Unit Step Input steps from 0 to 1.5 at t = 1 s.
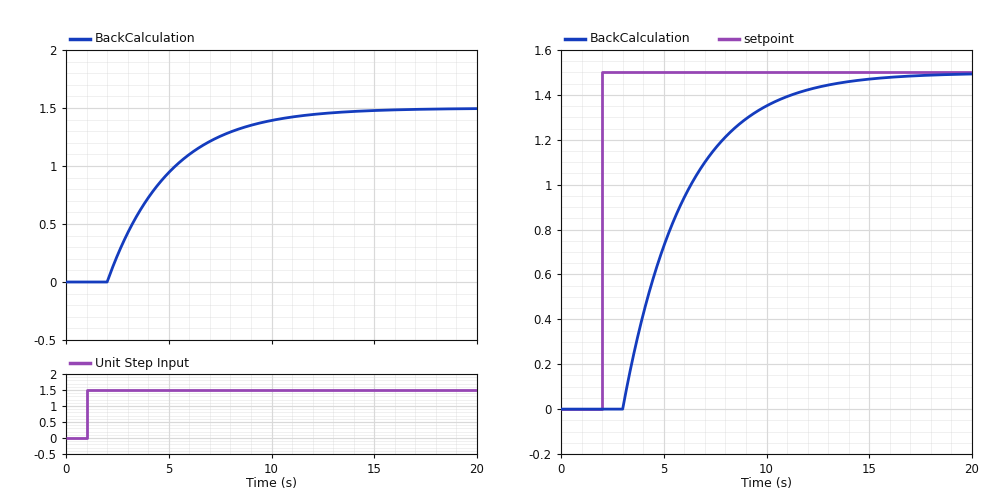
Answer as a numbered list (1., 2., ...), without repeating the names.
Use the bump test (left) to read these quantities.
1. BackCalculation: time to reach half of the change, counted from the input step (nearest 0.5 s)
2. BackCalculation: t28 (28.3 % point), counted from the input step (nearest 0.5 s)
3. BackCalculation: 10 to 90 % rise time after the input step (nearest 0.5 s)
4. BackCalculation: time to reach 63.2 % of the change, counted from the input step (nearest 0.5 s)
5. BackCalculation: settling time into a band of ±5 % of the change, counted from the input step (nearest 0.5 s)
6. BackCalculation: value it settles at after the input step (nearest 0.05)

1. 3.0 s
2. 2.0 s
3. 6.5 s
4. 4.0 s
5. 10.0 s
6. 1.50
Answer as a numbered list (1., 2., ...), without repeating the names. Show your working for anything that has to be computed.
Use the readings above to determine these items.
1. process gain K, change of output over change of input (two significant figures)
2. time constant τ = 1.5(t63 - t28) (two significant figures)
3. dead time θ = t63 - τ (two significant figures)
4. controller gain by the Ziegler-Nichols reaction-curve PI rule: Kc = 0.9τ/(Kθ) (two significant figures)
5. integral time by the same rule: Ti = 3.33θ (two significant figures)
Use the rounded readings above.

1. (1.5 - 0) / 1.5 = 1.0
2. 1.5 × (4 - 2) = 3.0 s
3. 4 - 3 = 1.0 s
4. 0.9 × 3 / (1 × 1) = 2.7
5. 3.33 × 1 = 3.3 s
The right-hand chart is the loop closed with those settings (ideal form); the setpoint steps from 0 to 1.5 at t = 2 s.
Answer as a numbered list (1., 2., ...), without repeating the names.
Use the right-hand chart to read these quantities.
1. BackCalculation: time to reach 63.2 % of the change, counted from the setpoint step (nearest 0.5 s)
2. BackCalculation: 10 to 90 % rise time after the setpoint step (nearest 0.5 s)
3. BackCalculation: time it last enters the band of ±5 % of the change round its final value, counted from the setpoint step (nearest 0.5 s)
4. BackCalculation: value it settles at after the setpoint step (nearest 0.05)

1. 4.0 s
2. 6.5 s
3. 10.0 s
4. 1.50
